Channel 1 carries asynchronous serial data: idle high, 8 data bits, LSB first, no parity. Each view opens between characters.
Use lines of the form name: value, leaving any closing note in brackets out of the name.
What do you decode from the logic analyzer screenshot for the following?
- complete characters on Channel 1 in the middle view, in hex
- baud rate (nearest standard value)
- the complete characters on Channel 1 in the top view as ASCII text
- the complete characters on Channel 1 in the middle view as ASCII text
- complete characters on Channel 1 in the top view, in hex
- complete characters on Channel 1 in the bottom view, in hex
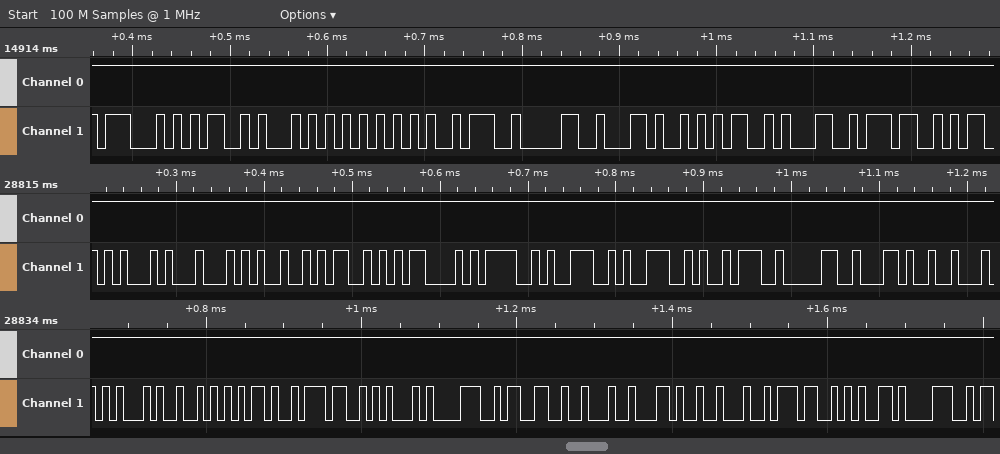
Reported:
complete characters on Channel 1 in the middle view, in hex: 45, 44, 49, 53, 43, 4F, 4E, 4E, 3A, 30, 2C
baud rate: 115200 baud
the complete characters on Channel 1 in the top view as ASCII text: "GMTU:0,517"
the complete characters on Channel 1 in the middle view as ASCII text: "EDISCONN:0,"
complete characters on Channel 1 in the top view, in hex: 47, 4D, 54, 55, 3A, 30, 2C, 35, 31, 37
complete characters on Channel 1 in the bottom view, in hex: 45, 52, 2D, 37, 45, 38, 33, 22, 2C, 22, 37, 65, 38
